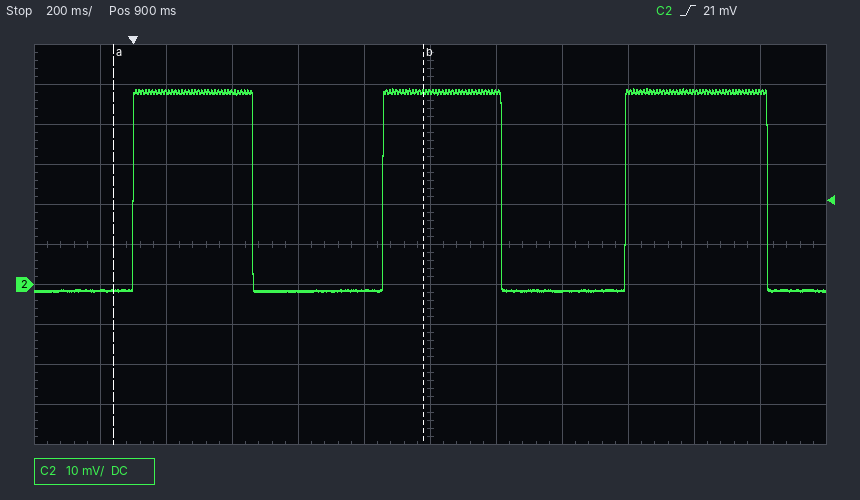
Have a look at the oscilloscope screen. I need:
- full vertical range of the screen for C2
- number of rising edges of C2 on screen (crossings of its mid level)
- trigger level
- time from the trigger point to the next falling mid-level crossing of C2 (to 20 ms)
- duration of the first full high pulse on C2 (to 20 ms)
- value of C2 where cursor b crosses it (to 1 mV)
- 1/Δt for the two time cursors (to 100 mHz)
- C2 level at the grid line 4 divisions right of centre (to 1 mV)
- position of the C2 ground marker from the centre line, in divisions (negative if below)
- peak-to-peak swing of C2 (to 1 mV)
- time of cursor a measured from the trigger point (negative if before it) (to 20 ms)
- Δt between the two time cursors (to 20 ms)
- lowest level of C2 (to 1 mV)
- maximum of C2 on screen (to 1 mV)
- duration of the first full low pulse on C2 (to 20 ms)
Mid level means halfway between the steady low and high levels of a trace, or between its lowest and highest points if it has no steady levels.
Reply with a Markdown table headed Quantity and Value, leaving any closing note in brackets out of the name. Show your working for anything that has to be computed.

| Quantity | Value |
|---|---|
| full vertical range of the screen for C2 | 100 mV |
| number of rising edges of C2 on screen | 3 |
| trigger level | 21 mV |
| time from the trigger point to the next falling mid-level crossing of C2 | 360 ms |
| duration of the first full high pulse on C2 | 360 ms |
| value of C2 where cursor b crosses it | 48 mV |
| 1/Δt for the two time cursors | 1 / 940 ms ≈ 1.1 Hz |
| C2 level at the grid line 4 divisions right of centre | 48 mV |
| position of the C2 ground marker from the centre line, in divisions | -1.0 div |
| peak-to-peak swing of C2 | 49 mV − (-2 mV) = 51 mV |
| time of cursor a measured from the trigger point (negative if before it) | -60 ms |
| Δt between the two time cursors | 940 ms |
| lowest level of C2 | -2 mV |
| maximum of C2 on screen | 49 mV |
| duration of the first full low pulse on C2 | 400 ms |
